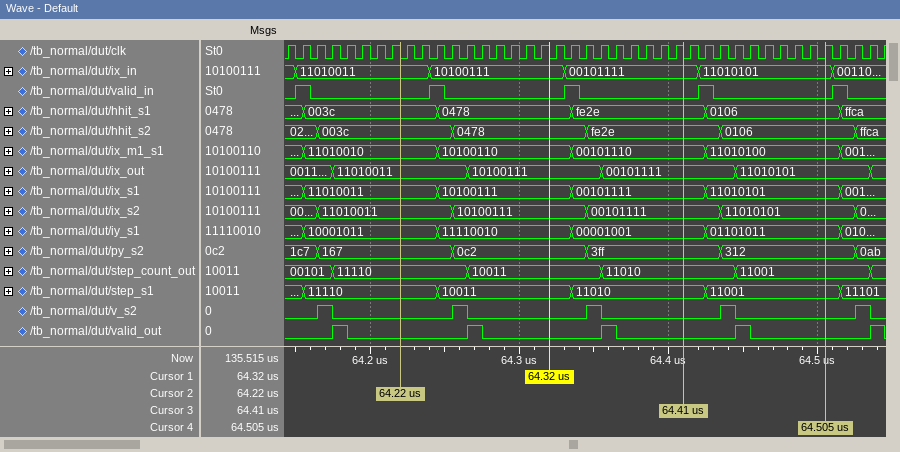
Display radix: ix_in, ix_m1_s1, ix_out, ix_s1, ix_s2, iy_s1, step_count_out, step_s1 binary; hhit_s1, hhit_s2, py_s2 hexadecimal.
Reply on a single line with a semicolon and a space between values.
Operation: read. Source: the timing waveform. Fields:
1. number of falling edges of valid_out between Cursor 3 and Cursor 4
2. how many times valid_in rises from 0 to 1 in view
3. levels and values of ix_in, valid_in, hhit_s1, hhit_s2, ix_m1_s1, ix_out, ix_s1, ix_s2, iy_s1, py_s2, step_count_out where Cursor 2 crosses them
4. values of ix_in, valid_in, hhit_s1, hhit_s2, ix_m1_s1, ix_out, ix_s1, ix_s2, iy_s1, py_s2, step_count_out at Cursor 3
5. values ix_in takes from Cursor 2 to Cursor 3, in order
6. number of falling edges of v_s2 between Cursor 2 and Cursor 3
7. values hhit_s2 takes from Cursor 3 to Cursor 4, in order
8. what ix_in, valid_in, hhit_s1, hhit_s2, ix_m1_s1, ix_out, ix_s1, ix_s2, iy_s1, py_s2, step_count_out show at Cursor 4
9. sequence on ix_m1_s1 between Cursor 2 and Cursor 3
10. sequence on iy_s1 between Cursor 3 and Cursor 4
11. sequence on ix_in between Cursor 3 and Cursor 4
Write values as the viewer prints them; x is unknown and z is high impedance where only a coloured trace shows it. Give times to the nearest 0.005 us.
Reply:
1; 5; ix_in=11010011, valid_in=0, hhit_s1=003c, hhit_s2=003c, ix_m1_s1=11010010, ix_out=11010011, ix_s1=11010011, ix_s2=11010011, iy_s1=10001011, py_s2=167, step_count_out=11110; ix_in=00101111, valid_in=0, hhit_s1=fe2e, hhit_s2=fe2e, ix_m1_s1=00101110, ix_out=00101111, ix_s1=00101111, ix_s2=00101111, iy_s1=00001001, py_s2=3ff, step_count_out=11010; 11010011, 10100111, 00101111; 2; fe2e, 0106; ix_in=11010101, valid_in=0, hhit_s1=0106, hhit_s2=0106, ix_m1_s1=11010100, ix_out=11010101, ix_s1=11010101, ix_s2=11010101, iy_s1=01101011, py_s2=312, step_count_out=11001; 11010010, 10100110, 00101110; 00001001, 01101011; 00101111, 11010101
